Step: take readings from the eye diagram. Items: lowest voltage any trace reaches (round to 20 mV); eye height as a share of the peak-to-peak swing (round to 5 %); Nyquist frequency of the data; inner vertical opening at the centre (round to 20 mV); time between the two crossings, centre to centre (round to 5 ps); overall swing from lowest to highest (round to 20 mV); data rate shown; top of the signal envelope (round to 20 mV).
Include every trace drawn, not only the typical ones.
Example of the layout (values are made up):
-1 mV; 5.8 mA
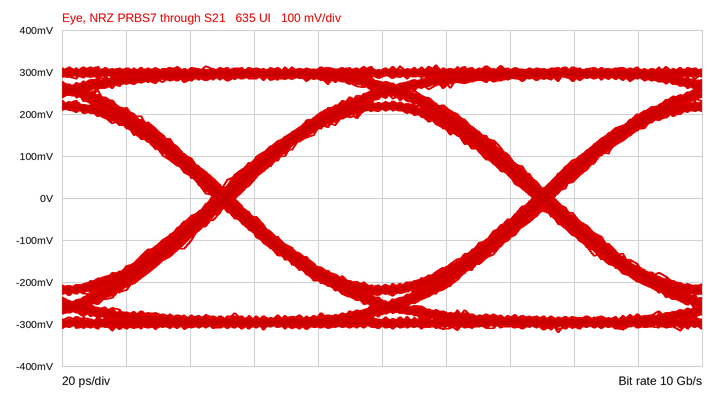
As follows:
-320 mV; 65 %; 5 GHz; 420 mV; 100 ps; 640 mV; 10 Gb/s; 320 mV
